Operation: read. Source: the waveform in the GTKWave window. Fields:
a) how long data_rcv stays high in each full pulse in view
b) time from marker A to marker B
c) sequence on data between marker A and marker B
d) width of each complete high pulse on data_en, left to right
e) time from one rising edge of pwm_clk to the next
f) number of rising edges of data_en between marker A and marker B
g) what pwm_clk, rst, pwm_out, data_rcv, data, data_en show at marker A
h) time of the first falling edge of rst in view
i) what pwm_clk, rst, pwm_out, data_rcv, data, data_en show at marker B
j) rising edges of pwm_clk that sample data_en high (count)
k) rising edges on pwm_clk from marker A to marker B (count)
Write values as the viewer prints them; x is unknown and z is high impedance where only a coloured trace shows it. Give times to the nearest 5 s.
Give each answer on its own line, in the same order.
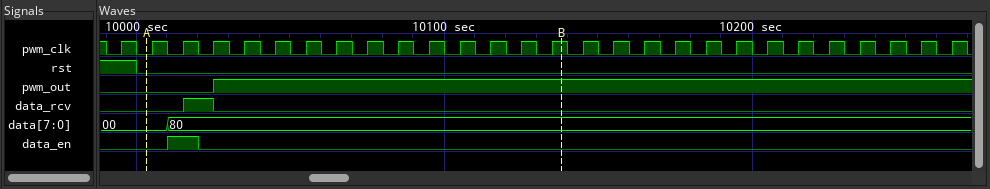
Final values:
10 s
135 s
00, 80
10 s
10 s
1
pwm_clk=0, rst=0, pwm_out=0, data_rcv=0, data=00, data_en=0
10000 s
pwm_clk=1, rst=0, pwm_out=1, data_rcv=0, data=80, data_en=0
1
14
